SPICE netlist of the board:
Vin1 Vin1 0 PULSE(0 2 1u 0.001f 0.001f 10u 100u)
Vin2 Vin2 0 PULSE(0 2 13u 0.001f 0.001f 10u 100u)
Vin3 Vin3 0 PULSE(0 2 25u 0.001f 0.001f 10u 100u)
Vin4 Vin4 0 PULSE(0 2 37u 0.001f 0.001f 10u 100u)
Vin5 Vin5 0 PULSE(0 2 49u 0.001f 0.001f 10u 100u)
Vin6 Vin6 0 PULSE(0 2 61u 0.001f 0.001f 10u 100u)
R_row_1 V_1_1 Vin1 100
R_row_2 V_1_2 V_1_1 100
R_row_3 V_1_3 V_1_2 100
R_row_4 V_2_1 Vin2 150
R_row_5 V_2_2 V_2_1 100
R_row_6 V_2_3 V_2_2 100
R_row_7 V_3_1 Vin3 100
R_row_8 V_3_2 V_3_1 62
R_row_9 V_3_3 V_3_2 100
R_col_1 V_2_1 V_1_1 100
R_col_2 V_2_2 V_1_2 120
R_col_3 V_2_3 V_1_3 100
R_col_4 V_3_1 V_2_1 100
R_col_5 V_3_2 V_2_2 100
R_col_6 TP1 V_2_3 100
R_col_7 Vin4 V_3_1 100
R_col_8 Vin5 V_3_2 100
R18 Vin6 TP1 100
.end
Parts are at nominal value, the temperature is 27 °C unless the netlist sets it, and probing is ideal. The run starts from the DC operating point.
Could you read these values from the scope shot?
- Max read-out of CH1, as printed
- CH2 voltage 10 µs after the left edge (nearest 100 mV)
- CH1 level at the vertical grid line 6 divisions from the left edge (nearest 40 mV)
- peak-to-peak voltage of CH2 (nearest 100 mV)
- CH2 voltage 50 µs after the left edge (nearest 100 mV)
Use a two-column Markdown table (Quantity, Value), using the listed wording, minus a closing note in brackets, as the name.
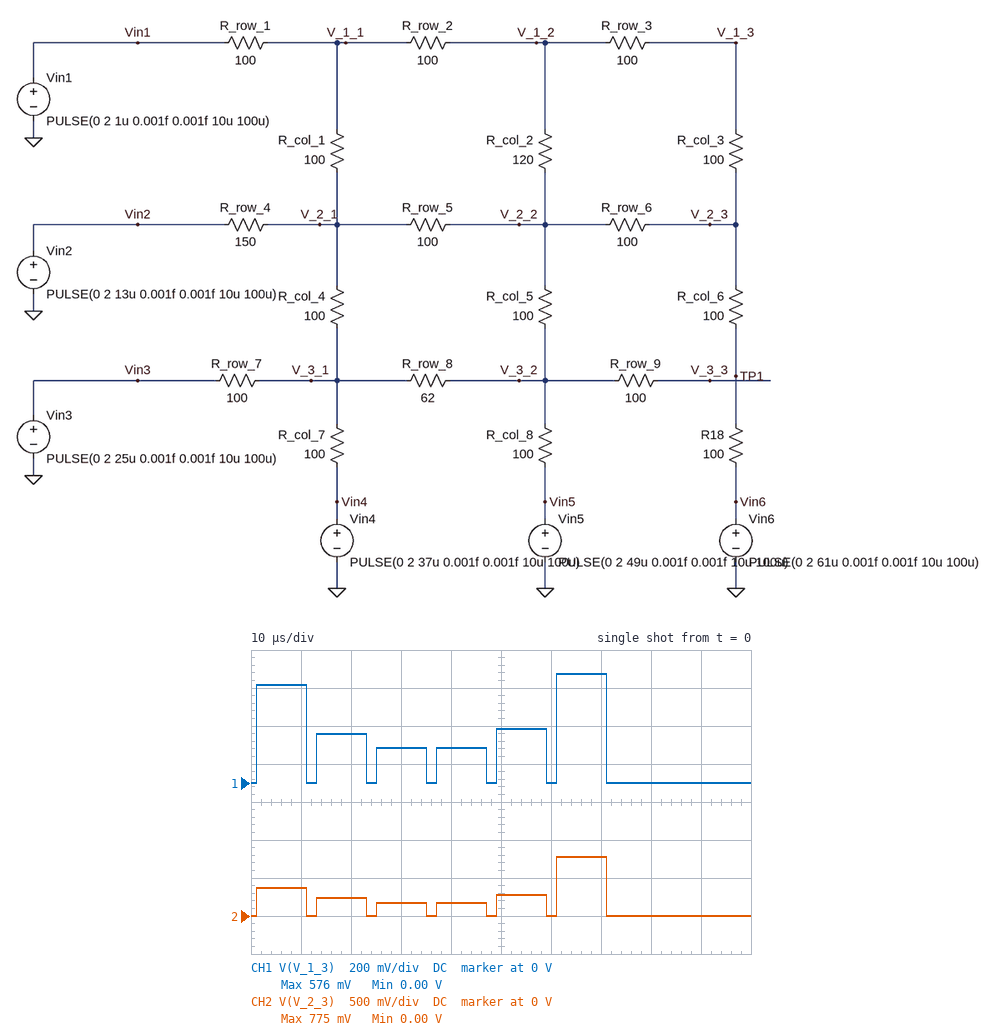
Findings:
| Quantity | Value |
|---|---|
| Max read-out of CH1, as printed | 576 mV |
| CH2 voltage 10 µs after the left edge | 400 mV |
| CH1 level at the vertical grid line 6 divisions from the left edge | 0 V |
| peak-to-peak voltage of CH2 | 800 mV |
| CH2 voltage 50 µs after the left edge | 300 mV |
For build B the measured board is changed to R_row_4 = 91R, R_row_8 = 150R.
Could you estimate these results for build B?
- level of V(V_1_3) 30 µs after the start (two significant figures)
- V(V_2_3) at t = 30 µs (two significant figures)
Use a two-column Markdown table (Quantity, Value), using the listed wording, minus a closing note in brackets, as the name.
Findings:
| Quantity | Value |
|---|---|
| level of V(V_1_3) 30 µs after the start | 140 mV |
| V(V_2_3) at t = 30 µs | 130 mV |
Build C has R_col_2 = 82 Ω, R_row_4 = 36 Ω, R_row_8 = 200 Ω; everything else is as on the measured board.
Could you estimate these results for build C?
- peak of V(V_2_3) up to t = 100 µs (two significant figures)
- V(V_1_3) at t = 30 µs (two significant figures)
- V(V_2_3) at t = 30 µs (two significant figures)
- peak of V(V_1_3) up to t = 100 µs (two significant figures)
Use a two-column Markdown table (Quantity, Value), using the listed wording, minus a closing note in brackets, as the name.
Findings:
| Quantity | Value |
|---|---|
| peak of V(V_2_3) up to t = 100 µs | 750 mV |
| V(V_1_3) at t = 30 µs | 99 mV |
| V(V_2_3) at t = 30 µs | 92 mV |
| peak of V(V_1_3) up to t = 100 µs | 560 mV |
